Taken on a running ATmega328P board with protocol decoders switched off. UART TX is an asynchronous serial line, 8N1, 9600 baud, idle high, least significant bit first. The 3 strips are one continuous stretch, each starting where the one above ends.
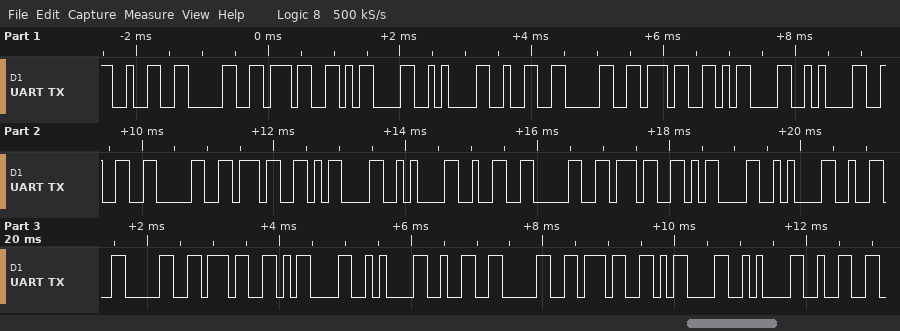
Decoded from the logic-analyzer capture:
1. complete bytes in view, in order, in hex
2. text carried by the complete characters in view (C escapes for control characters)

32 30 37 0D 0A 32 30 37 0D 0A 32 30 37 0D 0A 32 30 37 0D 0A 32 30 37 0D 0A 32 30 37 0D 0A 32
"207\r\n207\r\n207\r\n207\r\n207\r\n207\r\n2"
